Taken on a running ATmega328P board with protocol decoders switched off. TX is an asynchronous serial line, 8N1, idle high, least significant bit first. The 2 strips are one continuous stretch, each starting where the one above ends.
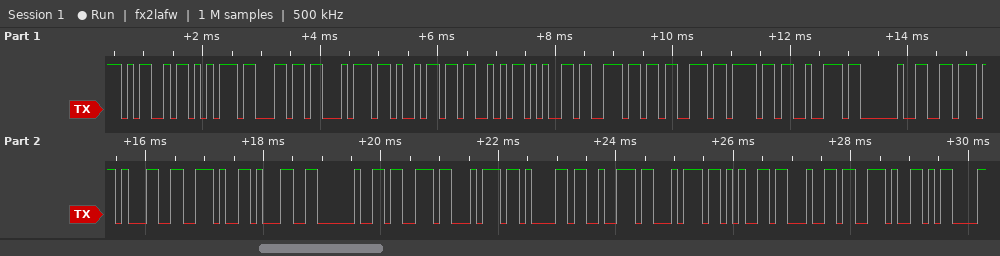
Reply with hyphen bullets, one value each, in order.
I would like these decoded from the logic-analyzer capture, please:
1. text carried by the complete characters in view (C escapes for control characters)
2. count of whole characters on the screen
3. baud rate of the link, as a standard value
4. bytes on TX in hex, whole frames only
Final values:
- "MultiSensor v1.1 started.\r"
- 26
- 9600 baud
- 4D 75 6C 74 69 53 65 6E 73 6F 72 20 76 31 2E 31 20 73 74 61 72 74 65 64 2E 0D
